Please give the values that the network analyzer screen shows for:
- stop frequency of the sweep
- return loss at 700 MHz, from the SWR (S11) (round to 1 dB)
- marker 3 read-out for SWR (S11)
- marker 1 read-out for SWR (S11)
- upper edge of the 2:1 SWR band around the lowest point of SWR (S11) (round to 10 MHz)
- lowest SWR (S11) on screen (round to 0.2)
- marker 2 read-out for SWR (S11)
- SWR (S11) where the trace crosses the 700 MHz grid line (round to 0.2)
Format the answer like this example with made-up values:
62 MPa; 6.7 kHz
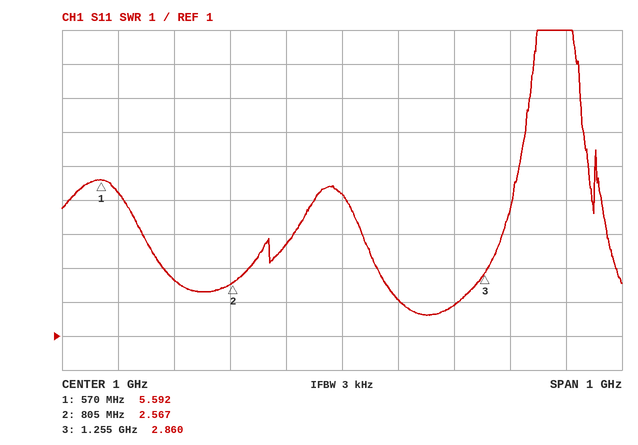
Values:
1.5 GHz; 7 dB; 2.860; 5.592; 1.21 GHz; 1.6; 2.567; 2.6
